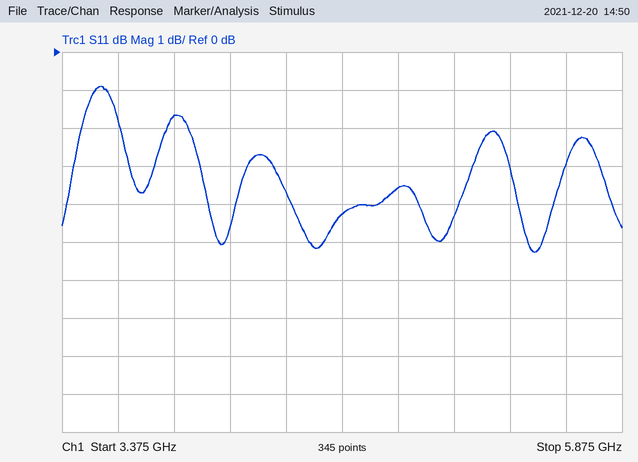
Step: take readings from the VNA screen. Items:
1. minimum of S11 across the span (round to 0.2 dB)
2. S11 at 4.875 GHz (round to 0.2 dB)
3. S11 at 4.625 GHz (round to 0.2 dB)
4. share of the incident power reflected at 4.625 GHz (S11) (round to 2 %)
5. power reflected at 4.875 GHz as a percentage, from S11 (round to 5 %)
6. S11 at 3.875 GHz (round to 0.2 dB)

-5.2 dB
-3.6 dB
-4.2 dB
38 %
45 %
-1.6 dB
